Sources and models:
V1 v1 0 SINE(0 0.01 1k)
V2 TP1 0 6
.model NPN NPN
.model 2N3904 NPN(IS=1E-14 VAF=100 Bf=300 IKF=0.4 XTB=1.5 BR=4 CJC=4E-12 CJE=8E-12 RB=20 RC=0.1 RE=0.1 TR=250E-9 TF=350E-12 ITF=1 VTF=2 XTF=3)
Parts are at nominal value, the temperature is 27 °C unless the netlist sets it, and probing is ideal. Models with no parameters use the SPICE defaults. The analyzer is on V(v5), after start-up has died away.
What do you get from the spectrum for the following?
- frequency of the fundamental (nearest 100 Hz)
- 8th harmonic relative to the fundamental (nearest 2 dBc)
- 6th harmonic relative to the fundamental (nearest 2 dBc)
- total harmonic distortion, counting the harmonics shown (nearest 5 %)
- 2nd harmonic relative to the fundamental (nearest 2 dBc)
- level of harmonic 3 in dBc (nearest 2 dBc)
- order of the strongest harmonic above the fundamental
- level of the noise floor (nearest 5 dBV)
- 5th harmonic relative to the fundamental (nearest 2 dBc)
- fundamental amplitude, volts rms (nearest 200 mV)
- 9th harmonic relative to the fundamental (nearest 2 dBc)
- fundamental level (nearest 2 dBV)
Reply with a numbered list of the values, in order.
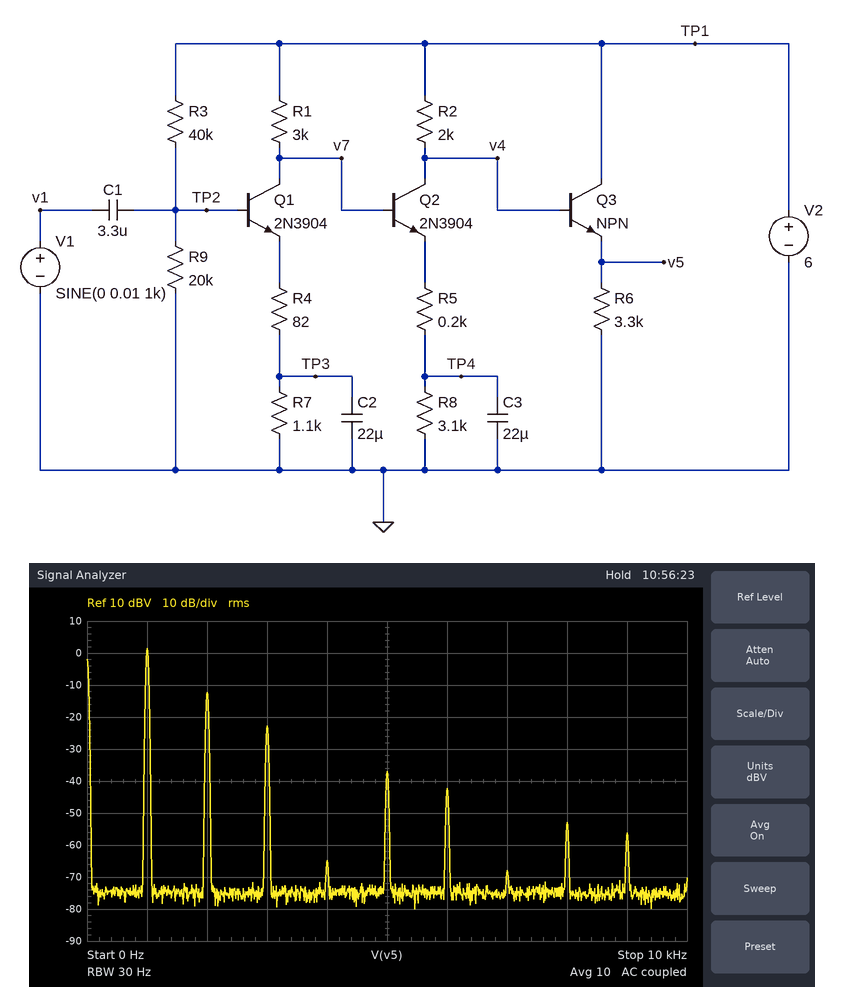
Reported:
1. 1.0 kHz
2. -54 dBc
3. -44 dBc
4. 20 %
5. -14 dBc
6. -24 dBc
7. 2
8. -75 dBV
9. -38 dBc
10. 1.2 V
11. -58 dBc
12. 2 dBV
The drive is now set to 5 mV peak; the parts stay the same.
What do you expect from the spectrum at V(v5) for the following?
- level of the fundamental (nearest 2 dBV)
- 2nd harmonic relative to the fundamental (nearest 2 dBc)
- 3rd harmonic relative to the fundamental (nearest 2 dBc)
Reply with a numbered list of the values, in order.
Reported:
1. -2 dBV
2. -26 dBc
3. -38 dBc
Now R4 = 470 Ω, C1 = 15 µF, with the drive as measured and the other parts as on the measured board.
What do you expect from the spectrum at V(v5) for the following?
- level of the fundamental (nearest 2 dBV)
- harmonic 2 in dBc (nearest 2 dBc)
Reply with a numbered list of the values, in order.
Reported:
1. -10 dBV
2. -42 dBc
